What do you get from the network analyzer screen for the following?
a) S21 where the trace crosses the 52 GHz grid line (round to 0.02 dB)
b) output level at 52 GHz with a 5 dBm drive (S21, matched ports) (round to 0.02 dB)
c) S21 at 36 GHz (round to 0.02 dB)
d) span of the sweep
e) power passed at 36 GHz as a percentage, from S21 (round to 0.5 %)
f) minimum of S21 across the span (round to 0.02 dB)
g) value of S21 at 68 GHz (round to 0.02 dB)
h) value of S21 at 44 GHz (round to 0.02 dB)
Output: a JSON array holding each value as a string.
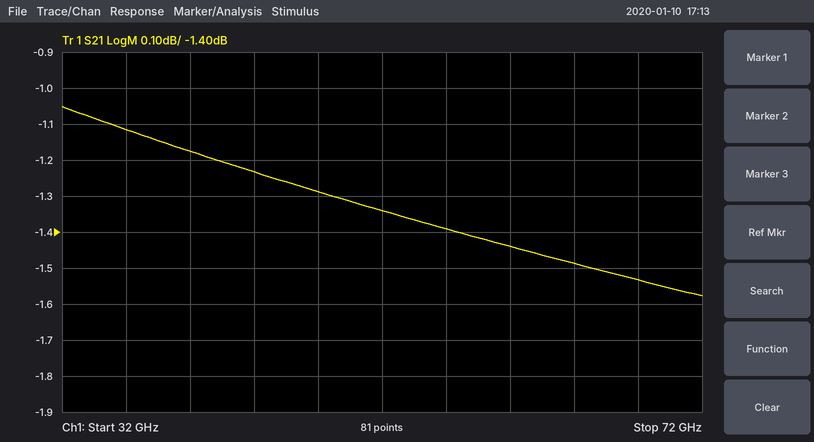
["-1.34 dB", "3.66 dBm", "-1.12 dB", "40 GHz", "77.5 %", "-1.58 dB", "-1.54 dB", "-1.24 dB"]
